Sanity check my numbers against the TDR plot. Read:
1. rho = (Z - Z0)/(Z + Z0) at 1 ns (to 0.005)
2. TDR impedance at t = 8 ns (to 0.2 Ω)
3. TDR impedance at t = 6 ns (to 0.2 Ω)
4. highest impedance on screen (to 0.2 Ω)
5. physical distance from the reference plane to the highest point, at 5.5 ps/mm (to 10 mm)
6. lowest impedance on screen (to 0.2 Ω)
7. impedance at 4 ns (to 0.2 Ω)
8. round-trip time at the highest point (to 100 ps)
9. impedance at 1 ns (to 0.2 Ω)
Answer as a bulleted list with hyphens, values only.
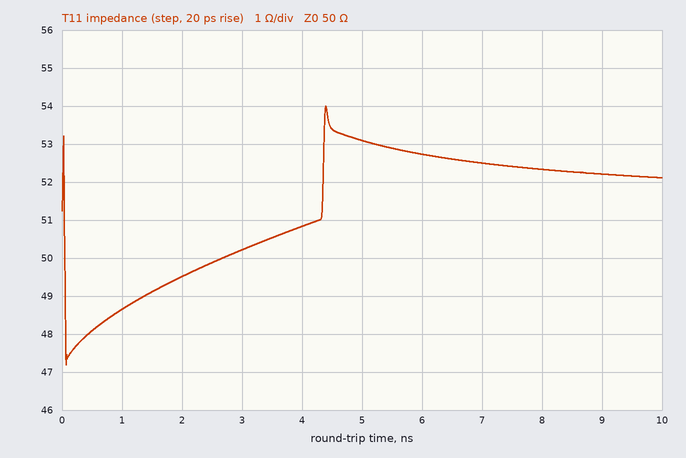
- -0.015
- 52.4 Ω
- 52.8 Ω
- 54.0 Ω
- 400 mm
- 47.2 Ω
- 50.8 Ω
- 4.4 ns
- 48.6 Ω
